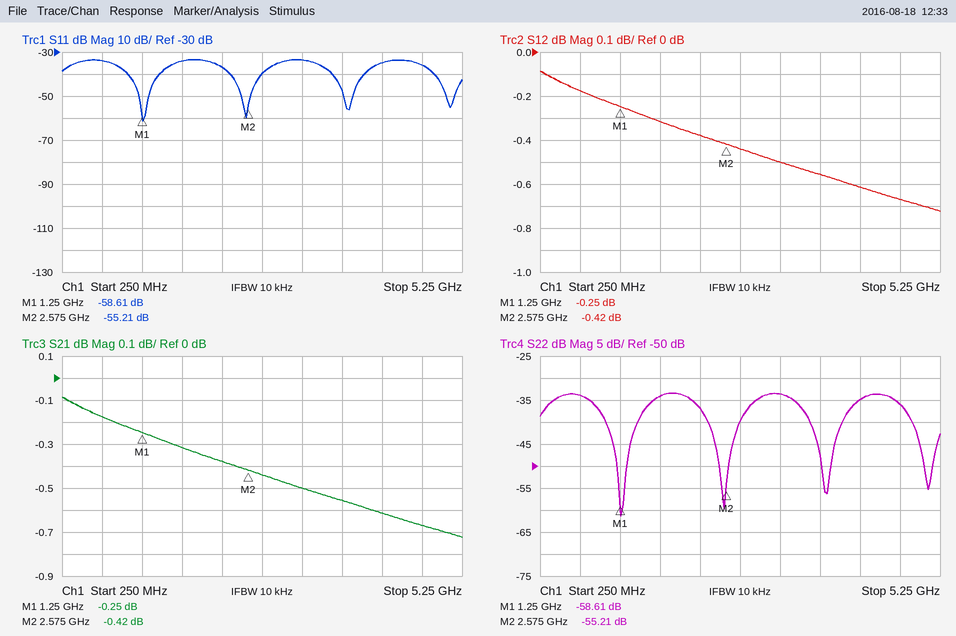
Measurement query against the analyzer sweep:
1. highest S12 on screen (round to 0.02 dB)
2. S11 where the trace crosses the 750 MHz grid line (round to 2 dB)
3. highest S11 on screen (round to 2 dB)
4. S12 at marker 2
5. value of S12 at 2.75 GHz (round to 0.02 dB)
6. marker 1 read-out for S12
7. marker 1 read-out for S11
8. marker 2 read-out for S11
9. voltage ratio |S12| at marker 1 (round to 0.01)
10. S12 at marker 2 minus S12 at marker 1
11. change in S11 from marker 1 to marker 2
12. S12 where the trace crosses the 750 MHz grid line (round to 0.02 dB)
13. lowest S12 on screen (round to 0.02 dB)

-0.08 dB
-34 dB
-34 dB
-0.42 dB
-0.44 dB
-0.25 dB
-58.61 dB
-55.21 dB
0.97
-0.17 dB
3.40 dB
-0.18 dB
-0.72 dB
